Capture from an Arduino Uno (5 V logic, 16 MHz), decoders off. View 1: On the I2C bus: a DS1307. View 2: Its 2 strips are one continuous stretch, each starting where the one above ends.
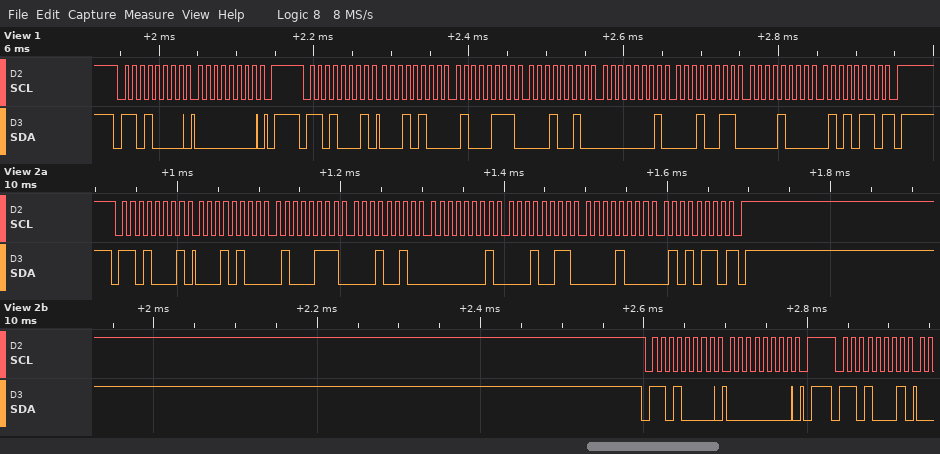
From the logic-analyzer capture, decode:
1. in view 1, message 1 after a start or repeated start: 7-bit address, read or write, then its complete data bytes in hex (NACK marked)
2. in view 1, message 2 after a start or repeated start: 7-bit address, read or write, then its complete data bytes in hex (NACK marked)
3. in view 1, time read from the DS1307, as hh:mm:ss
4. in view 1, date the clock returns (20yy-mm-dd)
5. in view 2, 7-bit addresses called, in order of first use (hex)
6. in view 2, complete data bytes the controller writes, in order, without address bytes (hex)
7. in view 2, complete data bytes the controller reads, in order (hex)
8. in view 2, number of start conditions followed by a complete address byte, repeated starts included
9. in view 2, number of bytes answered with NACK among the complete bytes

0x68 write: 00
0x68 read: 14 47 12 01 13 08 56 NACK
12:47:14
2056-08-13
0x68
00
14 47 12 01 13 08 56
3
1
